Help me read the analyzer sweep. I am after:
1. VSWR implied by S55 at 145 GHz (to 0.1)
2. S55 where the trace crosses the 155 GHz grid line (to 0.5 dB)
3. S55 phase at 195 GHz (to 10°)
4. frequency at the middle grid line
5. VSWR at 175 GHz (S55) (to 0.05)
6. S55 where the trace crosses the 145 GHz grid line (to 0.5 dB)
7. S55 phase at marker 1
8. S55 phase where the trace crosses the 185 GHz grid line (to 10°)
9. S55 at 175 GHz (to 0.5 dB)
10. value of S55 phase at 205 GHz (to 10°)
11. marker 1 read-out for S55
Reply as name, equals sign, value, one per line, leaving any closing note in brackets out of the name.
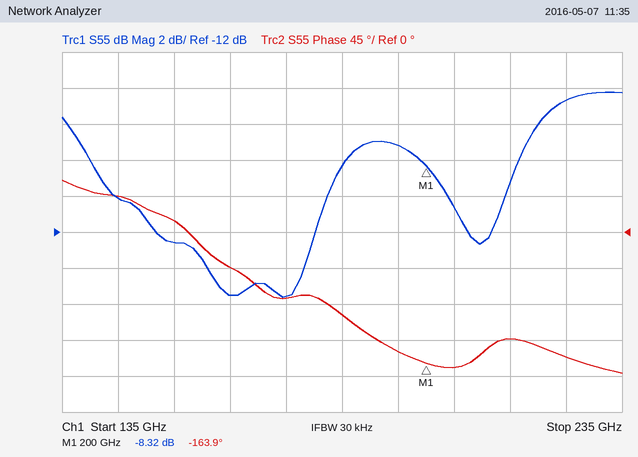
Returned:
VSWR implied by S55 at 145 GHz = 1.9
S55 where the trace crosses the 155 GHz grid line = -12.5 dB
S55 phase at 195 GHz = -150°
frequency at the middle grid line = 185 GHz
VSWR at 175 GHz (S55) = 1.40
S55 where the trace crosses the 145 GHz grid line = -10.0 dB
S55 phase at marker 1 = -163.9°
S55 phase where the trace crosses the 185 GHz grid line = -100°
S55 at 175 GHz = -15.5 dB
value of S55 phase at 205 GHz = -170°
marker 1 read-out for S55 = -8.32 dB
